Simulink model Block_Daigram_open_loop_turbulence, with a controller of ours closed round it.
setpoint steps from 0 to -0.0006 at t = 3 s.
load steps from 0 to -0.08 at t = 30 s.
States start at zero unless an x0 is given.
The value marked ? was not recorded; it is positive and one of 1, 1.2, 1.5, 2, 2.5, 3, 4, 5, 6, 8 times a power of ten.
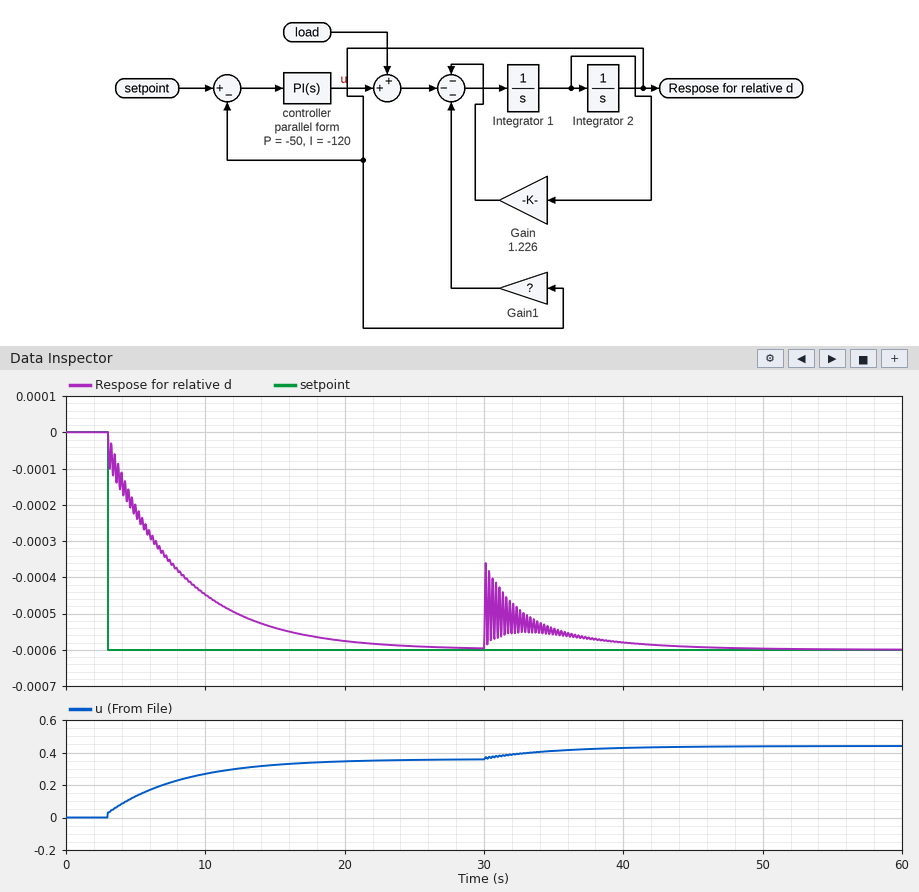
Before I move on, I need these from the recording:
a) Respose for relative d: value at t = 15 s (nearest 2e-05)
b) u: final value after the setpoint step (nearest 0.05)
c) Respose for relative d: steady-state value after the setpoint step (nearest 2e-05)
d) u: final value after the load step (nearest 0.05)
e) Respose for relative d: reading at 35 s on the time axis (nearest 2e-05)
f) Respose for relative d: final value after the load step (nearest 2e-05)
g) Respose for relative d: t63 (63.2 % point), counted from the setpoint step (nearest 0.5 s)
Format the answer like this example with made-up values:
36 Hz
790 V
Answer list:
-0.00054
0.35
-0.00060
0.45
-0.00054
-0.00060
5.0 s
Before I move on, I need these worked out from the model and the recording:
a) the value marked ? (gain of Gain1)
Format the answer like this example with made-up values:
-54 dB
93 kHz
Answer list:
600
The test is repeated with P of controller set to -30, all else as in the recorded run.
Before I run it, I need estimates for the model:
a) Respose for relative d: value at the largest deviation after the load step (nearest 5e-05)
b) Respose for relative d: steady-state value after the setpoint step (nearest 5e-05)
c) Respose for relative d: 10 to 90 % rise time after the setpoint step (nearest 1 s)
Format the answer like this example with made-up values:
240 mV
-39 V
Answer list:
-0.00035
-0.00060
12 s
